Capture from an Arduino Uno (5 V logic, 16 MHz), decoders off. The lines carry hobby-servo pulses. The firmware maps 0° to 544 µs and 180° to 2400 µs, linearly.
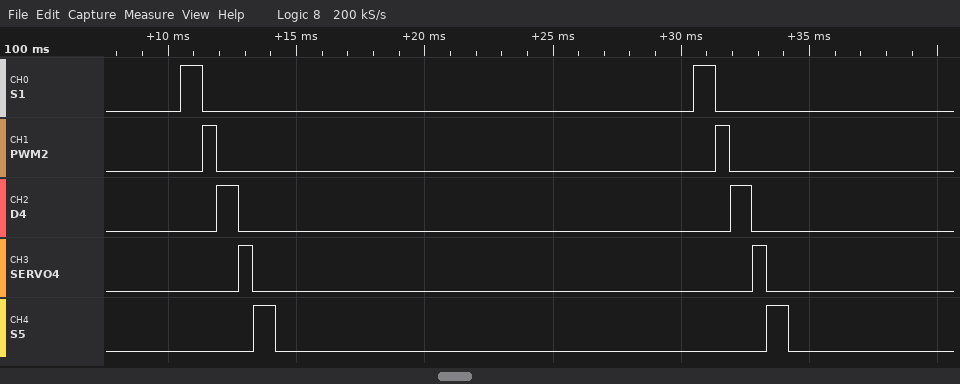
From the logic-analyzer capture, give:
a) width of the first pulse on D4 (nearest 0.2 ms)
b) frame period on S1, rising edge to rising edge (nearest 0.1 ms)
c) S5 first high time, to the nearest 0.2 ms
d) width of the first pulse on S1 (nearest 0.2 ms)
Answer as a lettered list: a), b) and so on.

a) 0.8 ms
b) 20.0 ms
c) 0.8 ms
d) 0.8 ms
